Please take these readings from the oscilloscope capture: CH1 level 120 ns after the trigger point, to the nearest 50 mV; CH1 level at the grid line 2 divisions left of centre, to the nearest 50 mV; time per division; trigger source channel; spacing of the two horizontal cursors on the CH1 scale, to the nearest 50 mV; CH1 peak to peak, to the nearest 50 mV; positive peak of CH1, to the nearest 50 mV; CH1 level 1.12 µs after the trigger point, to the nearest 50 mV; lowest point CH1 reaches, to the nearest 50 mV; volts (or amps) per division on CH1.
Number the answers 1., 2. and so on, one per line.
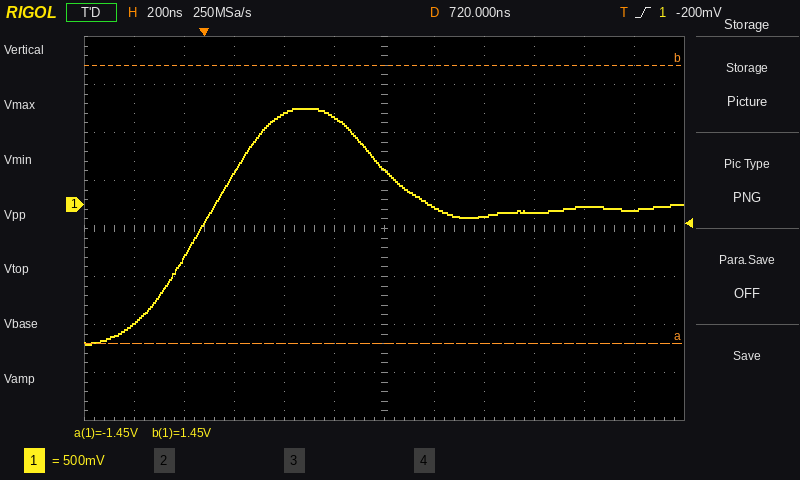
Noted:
1. 350 mV
2. 950 mV
3. 200 ns
4. CH1
5. 2.90 V
6. 2.45 V
7. 1.00 V
8. -100 mV
9. -1.45 V
10. 500 mV
